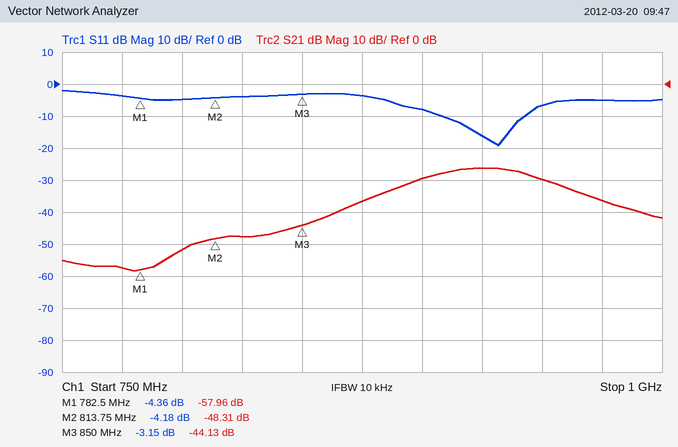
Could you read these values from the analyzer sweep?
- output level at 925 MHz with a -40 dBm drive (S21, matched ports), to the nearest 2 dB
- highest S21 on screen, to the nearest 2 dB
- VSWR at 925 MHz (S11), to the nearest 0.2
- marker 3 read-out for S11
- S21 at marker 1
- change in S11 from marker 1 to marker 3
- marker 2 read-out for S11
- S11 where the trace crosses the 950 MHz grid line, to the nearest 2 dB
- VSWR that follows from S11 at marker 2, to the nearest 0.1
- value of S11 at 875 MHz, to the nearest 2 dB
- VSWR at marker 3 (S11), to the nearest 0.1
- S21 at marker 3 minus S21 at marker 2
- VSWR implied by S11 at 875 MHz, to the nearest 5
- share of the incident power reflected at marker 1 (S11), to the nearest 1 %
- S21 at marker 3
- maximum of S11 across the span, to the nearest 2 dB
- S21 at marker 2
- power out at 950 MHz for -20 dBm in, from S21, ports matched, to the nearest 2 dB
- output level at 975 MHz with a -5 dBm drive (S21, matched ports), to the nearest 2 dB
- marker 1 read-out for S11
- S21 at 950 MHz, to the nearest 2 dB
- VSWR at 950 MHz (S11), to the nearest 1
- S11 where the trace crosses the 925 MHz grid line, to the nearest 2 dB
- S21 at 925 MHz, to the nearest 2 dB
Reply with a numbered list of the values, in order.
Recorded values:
1. -66 dBm
2. -26 dB
3. 1.4
4. -3.15 dB
5. -57.96 dB
6. 1.21 dB
7. -4.18 dB
8. -6 dB
9. 4.2
10. -4 dB
11. 5.6
12. 4.18 dB
13. 5
14. 37 %
15. -44.13 dB
16. -2 dB
17. -48.31 dB
18. -50 dBm
19. -42 dBm
20. -4.36 dB
21. -30 dB
22. 3
23. -16 dB
24. -26 dB
